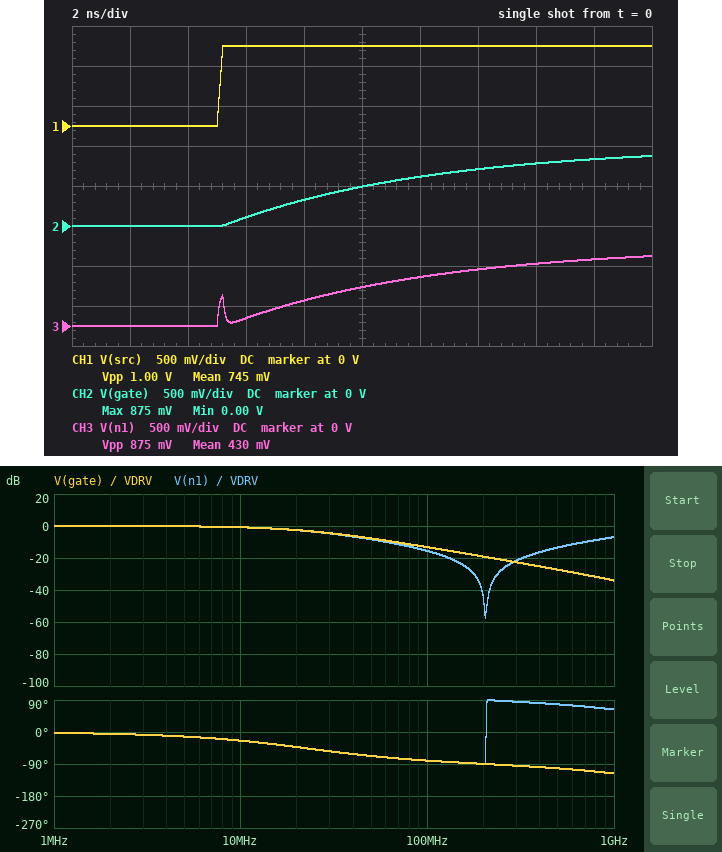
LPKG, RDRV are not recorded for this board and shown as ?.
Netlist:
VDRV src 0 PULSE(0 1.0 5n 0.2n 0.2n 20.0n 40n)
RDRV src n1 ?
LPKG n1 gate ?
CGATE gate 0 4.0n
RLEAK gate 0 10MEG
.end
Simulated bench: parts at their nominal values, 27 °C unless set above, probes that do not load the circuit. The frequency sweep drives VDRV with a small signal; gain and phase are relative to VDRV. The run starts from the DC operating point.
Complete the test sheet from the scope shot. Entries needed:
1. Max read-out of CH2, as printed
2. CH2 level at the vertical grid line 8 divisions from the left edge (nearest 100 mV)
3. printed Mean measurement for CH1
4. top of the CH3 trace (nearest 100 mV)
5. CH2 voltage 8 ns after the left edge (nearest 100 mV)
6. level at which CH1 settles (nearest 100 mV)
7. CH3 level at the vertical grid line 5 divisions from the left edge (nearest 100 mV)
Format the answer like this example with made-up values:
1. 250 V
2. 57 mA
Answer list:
1. 875 mV
2. 800 mV
3. 745 mV
4. 900 mV
5. 300 mV
6. 1.0 V
7. 500 mV
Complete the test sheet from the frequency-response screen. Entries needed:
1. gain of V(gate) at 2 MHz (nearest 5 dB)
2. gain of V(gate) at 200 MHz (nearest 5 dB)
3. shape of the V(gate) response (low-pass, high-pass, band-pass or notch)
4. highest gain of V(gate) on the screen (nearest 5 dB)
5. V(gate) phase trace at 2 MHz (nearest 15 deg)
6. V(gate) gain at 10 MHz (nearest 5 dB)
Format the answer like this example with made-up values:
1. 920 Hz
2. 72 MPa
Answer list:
1. 0 dB
2. -20 dB
3. low-pass
4. 0 dB
5. 0 deg
6. 0 dB
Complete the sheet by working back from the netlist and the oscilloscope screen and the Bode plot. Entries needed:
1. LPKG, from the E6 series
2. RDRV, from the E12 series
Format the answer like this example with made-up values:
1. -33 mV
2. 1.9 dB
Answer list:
1. 150 pH
2. 1.8 Ω
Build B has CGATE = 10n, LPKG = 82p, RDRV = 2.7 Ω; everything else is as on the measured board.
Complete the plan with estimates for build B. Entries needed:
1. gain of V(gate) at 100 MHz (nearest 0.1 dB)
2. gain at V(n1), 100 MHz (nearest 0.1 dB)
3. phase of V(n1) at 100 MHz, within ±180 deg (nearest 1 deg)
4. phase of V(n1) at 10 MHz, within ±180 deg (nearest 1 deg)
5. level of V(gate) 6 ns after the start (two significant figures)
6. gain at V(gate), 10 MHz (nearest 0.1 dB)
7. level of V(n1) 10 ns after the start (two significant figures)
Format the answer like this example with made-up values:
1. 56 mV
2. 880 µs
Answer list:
1. -24.6 dB
2. -28.0 dB
3. -88 deg
4. -60 deg
5. 32 mV
6. -5.9 dB
7. 160 mV
